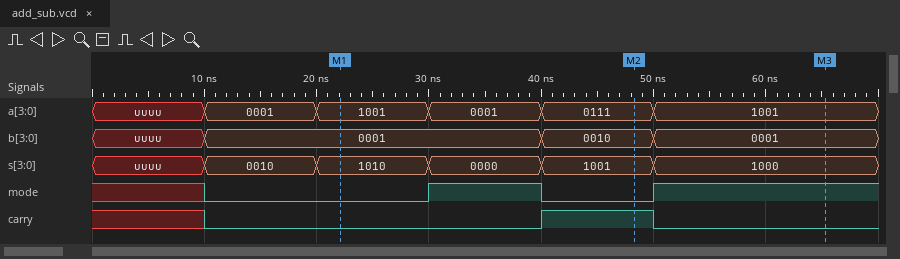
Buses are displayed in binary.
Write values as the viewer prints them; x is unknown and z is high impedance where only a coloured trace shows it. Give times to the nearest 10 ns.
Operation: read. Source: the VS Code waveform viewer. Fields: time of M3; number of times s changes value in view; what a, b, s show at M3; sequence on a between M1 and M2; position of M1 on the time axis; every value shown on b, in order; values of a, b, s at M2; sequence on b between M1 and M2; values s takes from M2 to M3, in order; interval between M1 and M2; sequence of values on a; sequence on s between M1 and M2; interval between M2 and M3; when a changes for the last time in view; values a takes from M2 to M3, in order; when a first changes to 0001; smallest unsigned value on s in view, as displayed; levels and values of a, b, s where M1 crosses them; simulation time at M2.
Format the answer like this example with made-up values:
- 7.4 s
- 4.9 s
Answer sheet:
- 70 ns
- 5
- a=1001, b=0001, s=1000
- 1001, 0001, 0111
- 20 ns
- uuuu, 0001, 0010, 0001
- a=0111, b=0010, s=1001
- 0001, 0010
- 1001, 1000
- 30 ns
- uuuu, 0001, 1001, 0001, 0111, 1001
- 1010, 0000, 1001
- 20 ns
- 50 ns
- 0111, 1001
- 10 ns
- 0000
- a=1001, b=0001, s=1010
- 50 ns
